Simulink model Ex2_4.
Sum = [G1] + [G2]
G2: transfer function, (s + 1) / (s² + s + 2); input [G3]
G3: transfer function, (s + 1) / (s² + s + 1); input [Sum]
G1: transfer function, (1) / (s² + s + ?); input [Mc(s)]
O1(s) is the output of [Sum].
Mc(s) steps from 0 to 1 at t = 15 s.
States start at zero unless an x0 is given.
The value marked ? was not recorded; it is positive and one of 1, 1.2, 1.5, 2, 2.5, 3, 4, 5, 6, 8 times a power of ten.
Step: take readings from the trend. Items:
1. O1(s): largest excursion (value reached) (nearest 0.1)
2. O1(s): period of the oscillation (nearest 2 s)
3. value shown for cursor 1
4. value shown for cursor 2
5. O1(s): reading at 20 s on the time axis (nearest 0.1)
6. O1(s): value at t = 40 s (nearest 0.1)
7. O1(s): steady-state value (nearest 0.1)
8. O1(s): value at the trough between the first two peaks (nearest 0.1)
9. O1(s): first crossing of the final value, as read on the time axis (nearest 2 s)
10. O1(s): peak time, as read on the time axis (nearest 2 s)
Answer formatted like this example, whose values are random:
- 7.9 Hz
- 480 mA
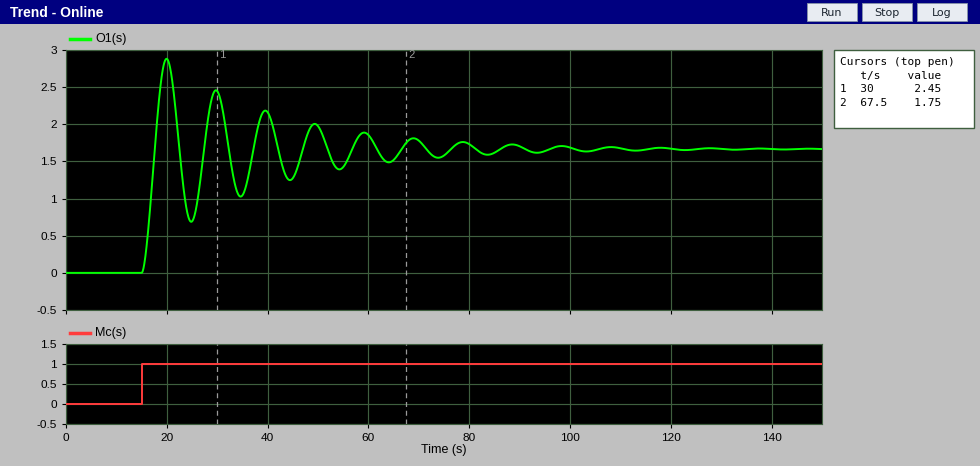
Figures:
- 2.9
- 10 s
- 2.45
- 1.75
- 2.9
- 2.2
- 1.7
- 0.7
- 18 s
- 20 s
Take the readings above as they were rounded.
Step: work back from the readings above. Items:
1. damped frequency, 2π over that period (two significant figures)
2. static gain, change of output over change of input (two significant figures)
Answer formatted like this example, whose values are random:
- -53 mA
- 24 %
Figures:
- 0.63 rad/s
- 1.7
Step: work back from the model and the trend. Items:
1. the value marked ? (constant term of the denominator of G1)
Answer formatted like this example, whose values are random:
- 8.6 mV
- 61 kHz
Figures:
- 1.2
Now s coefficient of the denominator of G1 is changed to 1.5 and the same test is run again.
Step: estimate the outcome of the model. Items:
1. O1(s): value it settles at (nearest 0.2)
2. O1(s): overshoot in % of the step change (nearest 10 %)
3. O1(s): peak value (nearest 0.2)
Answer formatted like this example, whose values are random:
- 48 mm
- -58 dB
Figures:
- 1.6
- 60 %
- 2.6
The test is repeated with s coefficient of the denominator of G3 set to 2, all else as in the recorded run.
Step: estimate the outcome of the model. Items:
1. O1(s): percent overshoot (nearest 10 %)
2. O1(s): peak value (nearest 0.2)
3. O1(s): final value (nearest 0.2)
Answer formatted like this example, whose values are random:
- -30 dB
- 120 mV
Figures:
- 20 %
- 2.0
- 1.6
